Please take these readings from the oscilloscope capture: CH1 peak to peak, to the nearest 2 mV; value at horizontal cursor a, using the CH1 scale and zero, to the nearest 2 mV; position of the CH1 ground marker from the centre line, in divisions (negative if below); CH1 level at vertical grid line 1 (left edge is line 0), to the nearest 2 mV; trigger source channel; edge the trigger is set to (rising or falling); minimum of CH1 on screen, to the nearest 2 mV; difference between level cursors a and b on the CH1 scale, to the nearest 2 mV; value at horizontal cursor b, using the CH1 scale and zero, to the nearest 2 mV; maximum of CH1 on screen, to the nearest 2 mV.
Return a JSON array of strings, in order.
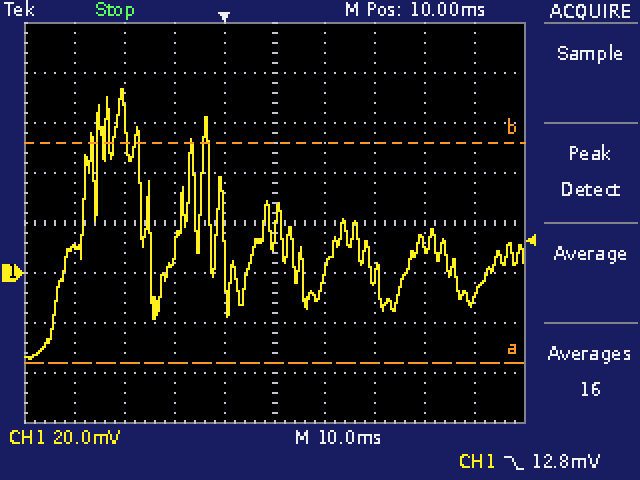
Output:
["108 mV", "-36 mV", "-1.0 div", "10 mV", "CH1", "falling", "-34 mV", "88 mV", "52 mV", "74 mV"]
